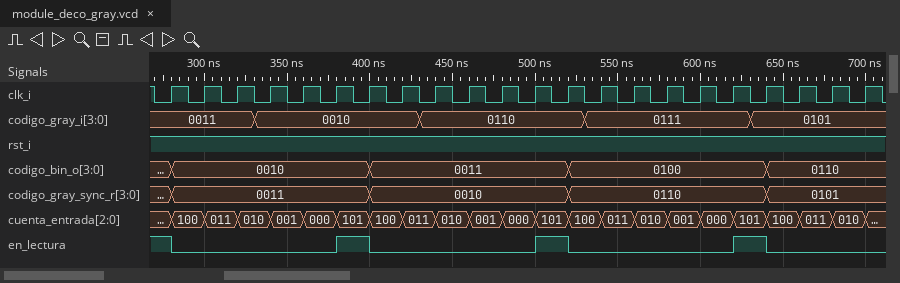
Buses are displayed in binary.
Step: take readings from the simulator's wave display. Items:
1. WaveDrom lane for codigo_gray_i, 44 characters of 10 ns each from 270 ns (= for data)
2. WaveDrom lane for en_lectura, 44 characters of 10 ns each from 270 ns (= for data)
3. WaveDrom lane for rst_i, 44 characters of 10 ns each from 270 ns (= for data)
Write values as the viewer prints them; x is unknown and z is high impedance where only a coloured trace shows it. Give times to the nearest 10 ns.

{name: 'codigo_gray_i', wave: '=.....=.........=.........=.........=.......', data: '0011 0010 0110 0111 0101'}
{name: 'en_lectura', wave: '10.........1.0.........1.0.........1.0......'}
{name: 'rst_i', wave: '1...........................................'}
